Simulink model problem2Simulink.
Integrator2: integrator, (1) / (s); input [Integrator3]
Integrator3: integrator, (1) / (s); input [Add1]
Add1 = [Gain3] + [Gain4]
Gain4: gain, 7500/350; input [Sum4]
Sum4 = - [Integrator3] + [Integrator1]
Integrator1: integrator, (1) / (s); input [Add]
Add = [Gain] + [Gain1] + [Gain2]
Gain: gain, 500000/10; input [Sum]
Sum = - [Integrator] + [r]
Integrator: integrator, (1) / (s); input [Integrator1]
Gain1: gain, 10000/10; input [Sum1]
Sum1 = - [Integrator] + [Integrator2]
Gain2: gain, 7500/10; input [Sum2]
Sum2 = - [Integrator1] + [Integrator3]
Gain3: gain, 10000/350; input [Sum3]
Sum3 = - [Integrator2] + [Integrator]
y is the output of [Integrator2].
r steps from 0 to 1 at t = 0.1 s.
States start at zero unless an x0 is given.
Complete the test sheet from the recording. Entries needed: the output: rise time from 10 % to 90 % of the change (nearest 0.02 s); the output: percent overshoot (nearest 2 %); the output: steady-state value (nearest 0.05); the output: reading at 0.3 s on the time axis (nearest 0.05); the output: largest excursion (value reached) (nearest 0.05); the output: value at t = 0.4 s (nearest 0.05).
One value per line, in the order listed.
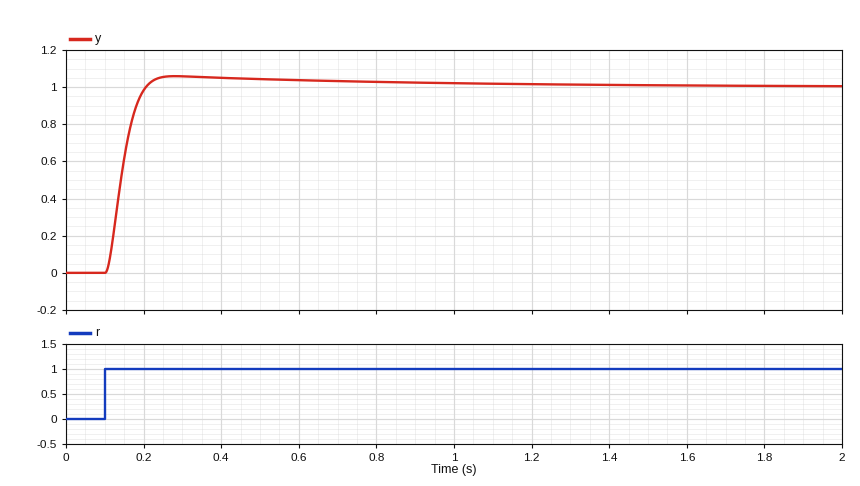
0.06 s
6 %
1.00
1.05
1.05
1.05
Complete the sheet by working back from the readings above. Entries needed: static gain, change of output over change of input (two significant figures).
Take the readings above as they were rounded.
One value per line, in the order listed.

1.0
